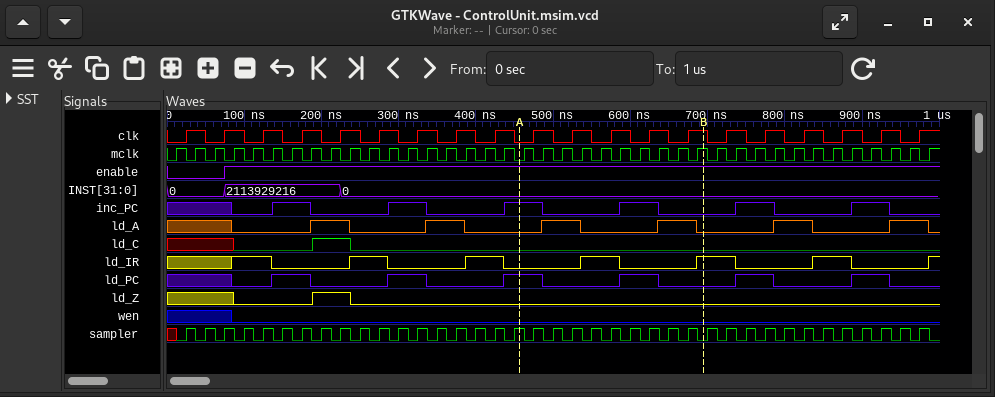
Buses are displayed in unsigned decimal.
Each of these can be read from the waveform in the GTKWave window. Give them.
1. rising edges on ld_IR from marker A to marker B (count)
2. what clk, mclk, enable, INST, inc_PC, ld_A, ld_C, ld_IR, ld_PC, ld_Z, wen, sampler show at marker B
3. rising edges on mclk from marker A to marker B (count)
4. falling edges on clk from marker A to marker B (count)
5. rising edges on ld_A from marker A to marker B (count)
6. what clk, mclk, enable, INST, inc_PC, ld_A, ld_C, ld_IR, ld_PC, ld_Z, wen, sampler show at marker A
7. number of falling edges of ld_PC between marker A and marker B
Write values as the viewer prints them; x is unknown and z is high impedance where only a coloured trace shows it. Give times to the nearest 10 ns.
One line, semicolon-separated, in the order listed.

2; clk=1, mclk=1, enable=1, INST=0, inc_PC=0, ld_A=0, ld_C=0, ld_IR=1, ld_PC=0, ld_Z=0, wen=0, sampler=0; 10; 4; 2; clk=0, mclk=0, enable=1, INST=0, inc_PC=1, ld_A=0, ld_C=0, ld_IR=0, ld_PC=1, ld_Z=0, wen=0, sampler=1; 2
